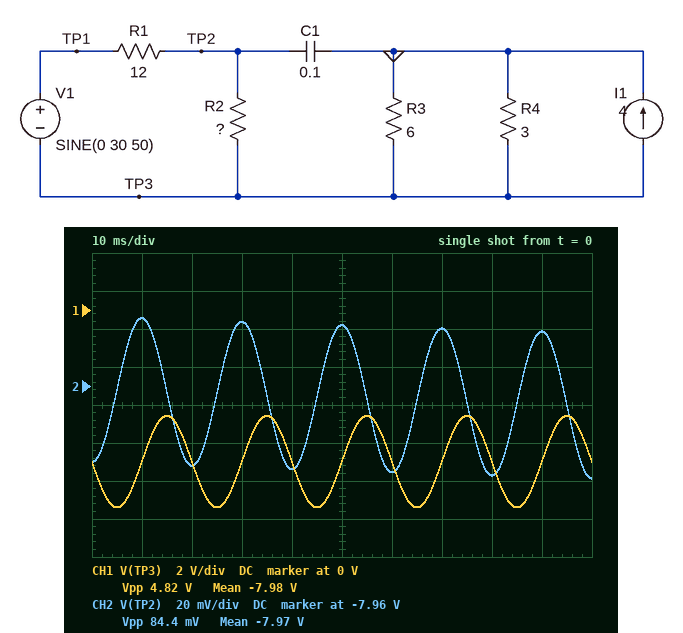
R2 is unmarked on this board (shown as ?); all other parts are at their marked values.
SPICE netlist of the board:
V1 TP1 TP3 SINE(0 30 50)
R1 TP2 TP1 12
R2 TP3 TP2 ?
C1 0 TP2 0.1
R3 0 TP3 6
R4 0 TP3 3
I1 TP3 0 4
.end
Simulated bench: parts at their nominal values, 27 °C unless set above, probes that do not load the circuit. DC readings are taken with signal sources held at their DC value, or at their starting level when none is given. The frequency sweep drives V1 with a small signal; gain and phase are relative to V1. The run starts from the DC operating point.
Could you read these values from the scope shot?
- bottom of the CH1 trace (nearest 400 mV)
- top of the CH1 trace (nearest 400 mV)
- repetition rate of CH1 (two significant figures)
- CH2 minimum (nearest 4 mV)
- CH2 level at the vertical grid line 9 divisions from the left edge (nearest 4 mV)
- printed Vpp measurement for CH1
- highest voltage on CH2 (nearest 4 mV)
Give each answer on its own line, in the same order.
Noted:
-10.4 V
-5.6 V
50 Hz
-8.008 V
-7.932 V
4.82 V
-7.924 V
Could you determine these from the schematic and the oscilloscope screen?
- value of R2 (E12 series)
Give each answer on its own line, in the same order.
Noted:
2.2 Ω
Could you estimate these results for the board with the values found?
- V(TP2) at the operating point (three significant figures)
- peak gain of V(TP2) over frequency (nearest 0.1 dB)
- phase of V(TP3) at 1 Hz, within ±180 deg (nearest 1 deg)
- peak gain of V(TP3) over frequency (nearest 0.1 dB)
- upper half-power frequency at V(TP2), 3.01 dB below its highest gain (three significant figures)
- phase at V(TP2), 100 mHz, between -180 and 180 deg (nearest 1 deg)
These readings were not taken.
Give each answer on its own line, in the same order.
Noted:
-8.00 V
-16.2 dB
-158 deg
-21.9 dB
412 mHz
-14 deg
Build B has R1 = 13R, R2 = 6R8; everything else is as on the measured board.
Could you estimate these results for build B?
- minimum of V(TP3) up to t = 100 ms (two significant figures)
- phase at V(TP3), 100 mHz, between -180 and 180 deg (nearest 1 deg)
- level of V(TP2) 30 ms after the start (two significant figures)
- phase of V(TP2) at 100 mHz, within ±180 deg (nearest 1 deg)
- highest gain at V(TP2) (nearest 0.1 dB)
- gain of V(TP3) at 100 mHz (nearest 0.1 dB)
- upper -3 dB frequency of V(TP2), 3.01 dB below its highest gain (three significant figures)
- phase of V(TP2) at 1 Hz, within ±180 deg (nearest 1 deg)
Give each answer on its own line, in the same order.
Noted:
-11 V
-112 deg
-7.9 V
-22 deg
-9.3 dB
-28.0 dB
246 mHz
-76 deg
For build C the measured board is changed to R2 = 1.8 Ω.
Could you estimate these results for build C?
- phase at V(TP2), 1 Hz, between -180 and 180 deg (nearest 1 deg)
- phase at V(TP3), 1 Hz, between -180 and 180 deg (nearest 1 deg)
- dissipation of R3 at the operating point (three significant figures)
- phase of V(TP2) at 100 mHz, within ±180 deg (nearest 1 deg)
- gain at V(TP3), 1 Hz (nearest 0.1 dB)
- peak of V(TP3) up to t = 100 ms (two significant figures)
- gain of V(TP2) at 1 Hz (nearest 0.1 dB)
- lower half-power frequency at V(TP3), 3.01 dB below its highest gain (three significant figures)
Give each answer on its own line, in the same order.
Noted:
-66 deg
-156 deg
10.7 W
-13 deg
-23.5 dB
-5.8 V
-25.5 dB
446 mHz
